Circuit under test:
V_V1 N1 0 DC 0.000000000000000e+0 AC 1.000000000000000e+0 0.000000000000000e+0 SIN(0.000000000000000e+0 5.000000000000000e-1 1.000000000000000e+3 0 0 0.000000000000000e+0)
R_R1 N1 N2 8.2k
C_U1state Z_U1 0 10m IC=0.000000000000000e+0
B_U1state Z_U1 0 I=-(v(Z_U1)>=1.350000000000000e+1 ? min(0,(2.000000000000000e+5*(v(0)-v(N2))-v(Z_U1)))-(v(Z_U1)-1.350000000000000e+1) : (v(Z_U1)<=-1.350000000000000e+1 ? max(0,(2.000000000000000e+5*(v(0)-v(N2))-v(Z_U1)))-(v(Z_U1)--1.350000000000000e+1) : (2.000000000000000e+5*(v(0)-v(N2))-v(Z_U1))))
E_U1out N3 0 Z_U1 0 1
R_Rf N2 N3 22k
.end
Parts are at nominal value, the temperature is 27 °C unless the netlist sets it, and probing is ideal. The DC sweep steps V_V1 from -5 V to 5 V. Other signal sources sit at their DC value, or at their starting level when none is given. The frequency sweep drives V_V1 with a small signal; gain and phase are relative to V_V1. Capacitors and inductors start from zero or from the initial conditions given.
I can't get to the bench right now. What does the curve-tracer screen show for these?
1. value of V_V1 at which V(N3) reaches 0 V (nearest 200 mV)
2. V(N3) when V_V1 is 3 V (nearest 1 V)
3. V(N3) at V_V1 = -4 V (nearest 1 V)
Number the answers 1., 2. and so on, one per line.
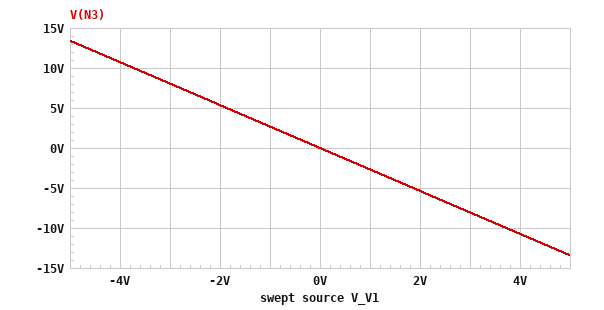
1. 0 V
2. -8 V
3. 11 V
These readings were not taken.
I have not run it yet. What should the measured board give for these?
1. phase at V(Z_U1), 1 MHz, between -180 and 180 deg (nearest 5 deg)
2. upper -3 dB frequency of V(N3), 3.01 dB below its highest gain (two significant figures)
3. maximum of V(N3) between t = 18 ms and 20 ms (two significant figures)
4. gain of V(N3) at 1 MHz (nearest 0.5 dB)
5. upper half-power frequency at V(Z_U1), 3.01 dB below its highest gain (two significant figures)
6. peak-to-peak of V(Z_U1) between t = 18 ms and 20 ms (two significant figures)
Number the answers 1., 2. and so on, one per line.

1. 130 deg
2. 860 kHz
3. 1.3 V
4. 5.0 dB
5. 860 kHz
6. 2.7 V
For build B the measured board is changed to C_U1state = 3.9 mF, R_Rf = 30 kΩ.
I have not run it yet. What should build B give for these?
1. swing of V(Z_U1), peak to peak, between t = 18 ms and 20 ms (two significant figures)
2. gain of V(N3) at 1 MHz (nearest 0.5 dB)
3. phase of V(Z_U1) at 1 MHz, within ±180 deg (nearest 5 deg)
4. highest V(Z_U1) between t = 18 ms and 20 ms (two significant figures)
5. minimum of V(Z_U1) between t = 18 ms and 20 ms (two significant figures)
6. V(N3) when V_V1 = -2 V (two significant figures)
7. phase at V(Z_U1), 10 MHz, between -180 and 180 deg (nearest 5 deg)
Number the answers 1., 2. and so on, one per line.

1. 3.7 V
2. 10.0 dB
3. 150 deg
4. 1.8 V
5. -1.8 V
6. 7.3 V
7. 100 deg
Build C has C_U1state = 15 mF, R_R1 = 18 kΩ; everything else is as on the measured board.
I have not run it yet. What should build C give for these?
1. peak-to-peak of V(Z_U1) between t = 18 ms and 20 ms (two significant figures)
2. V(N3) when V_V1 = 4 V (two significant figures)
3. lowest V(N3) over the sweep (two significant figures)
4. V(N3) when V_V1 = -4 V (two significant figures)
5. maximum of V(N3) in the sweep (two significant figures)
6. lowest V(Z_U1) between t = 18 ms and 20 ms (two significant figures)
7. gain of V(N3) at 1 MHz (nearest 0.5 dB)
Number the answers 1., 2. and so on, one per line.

1. 1.2 V
2. -4.9 V
3. -6.1 V
4. 4.9 V
5. 6.1 V
6. -610 mV
7. -1.5 dB
